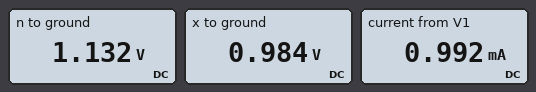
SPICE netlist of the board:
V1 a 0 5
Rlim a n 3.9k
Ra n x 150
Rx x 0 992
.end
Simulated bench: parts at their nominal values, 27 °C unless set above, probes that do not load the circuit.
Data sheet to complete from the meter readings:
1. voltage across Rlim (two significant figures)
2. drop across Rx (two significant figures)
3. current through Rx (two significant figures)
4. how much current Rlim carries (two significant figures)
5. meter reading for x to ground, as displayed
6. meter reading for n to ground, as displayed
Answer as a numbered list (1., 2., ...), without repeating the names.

1. 3.9 V
2. 980 mV
3. 990 µA
4. 990 µA
5. 0.984 V
6. 1.132 V
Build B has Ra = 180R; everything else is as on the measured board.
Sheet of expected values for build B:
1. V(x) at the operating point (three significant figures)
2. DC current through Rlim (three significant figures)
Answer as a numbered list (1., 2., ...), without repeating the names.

1. 978 mV
2. 986 µA
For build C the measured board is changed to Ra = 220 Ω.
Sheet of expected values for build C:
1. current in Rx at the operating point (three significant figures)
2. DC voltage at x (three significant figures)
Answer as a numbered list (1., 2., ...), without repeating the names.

1. 978 µA
2. 970 mV
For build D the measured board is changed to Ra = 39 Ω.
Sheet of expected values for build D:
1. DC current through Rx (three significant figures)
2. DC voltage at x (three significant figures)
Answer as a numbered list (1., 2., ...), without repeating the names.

1. 1.01 mA
2. 1.01 V
